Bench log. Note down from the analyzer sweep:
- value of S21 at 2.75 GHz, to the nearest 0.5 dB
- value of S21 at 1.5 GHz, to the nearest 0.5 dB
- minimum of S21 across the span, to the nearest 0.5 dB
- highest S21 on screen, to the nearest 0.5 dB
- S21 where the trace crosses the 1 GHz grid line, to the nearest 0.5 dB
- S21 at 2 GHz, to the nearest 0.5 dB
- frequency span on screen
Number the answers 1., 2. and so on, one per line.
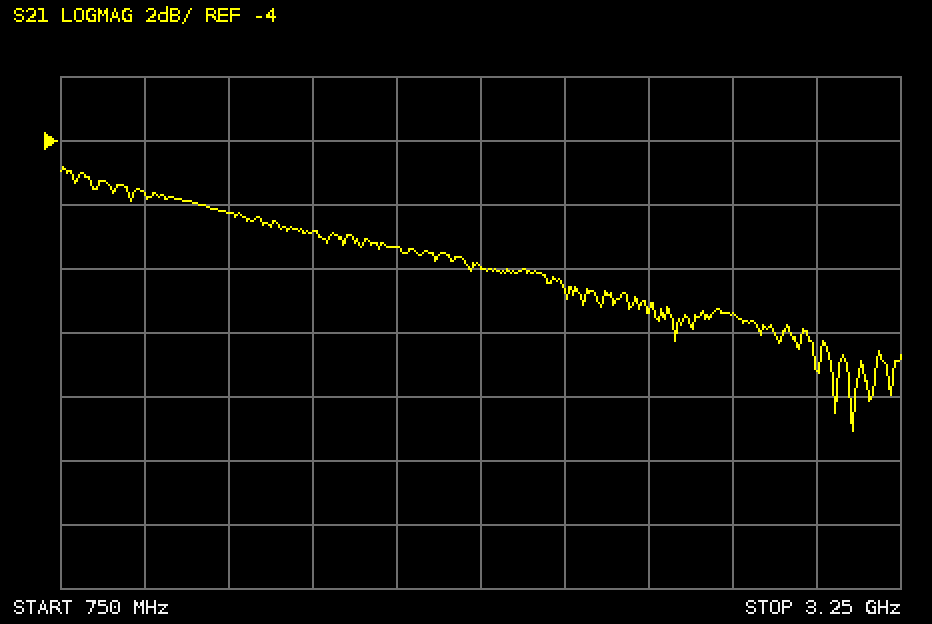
1. -9.5 dB
2. -7.0 dB
3. -13.0 dB
4. -5.0 dB
5. -5.5 dB
6. -8.0 dB
7. 2.5 GHz
